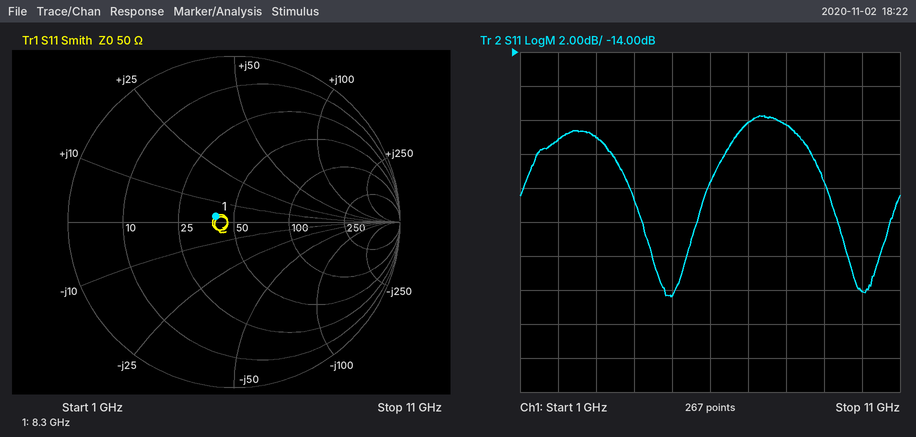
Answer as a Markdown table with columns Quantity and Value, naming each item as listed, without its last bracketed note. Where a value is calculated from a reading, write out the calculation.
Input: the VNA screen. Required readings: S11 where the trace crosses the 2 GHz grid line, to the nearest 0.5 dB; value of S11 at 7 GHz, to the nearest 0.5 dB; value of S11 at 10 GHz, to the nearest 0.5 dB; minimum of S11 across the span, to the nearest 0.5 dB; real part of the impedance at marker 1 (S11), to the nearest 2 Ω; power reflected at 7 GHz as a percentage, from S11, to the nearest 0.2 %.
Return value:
| Quantity | Value |
|---|---|
| S11 where the trace crosses the 2 GHz grid line, to the nearest 0.5 dB | -19.0 dB |
| value of S11 at 7 GHz, to the nearest 0.5 dB | -18.0 dB |
| value of S11 at 10 GHz, to the nearest 0.5 dB | -28.0 dB |
| minimum of S11 across the span, to the nearest 0.5 dB | -28.5 dB |
| real part of the impedance at marker 1 (S11), to the nearest 2 Ω | 40 Ω |
| power reflected at 7 GHz as a percentage, from S11, to the nearest 0.2 % | 10^(-18/10) ≈ 1.6 % |
